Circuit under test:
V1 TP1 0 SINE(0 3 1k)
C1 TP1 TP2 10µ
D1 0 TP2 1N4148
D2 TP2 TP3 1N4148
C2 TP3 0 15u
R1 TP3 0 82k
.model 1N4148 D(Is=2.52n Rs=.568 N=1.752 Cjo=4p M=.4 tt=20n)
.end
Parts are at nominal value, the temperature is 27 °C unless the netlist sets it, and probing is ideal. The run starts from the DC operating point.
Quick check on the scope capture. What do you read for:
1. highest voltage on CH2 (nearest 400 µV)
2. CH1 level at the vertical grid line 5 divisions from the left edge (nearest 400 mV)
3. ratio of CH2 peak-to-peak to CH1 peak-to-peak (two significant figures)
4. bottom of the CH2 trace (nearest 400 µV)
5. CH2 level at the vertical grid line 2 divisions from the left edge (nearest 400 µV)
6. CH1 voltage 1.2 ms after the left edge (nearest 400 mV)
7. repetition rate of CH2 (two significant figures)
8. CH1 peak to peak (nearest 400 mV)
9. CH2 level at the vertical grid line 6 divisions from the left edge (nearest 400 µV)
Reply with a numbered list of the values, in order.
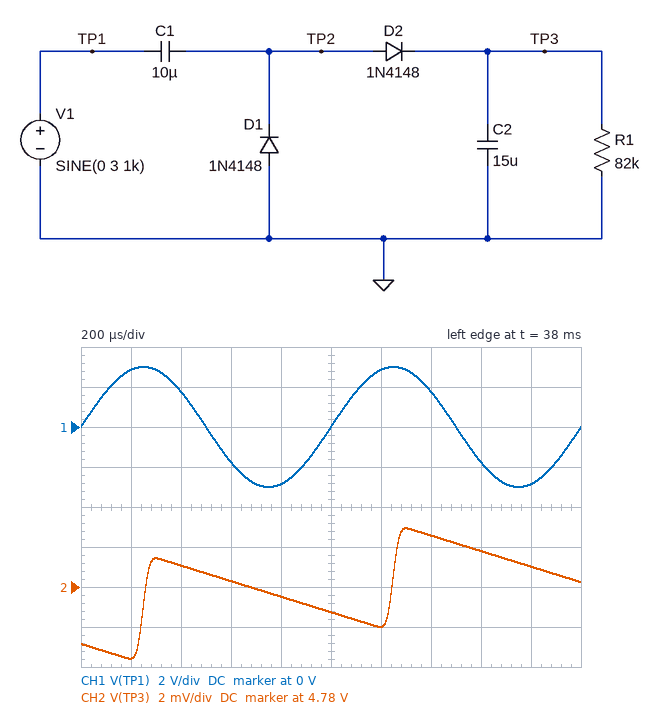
1. 4.7828 V
2. 0 V
3. 0.0011
4. 4.7764 V
5. 4.7812 V
6. 2.8 V
7. 1.0 kHz
8. 6.0 V
9. 4.7780 V
